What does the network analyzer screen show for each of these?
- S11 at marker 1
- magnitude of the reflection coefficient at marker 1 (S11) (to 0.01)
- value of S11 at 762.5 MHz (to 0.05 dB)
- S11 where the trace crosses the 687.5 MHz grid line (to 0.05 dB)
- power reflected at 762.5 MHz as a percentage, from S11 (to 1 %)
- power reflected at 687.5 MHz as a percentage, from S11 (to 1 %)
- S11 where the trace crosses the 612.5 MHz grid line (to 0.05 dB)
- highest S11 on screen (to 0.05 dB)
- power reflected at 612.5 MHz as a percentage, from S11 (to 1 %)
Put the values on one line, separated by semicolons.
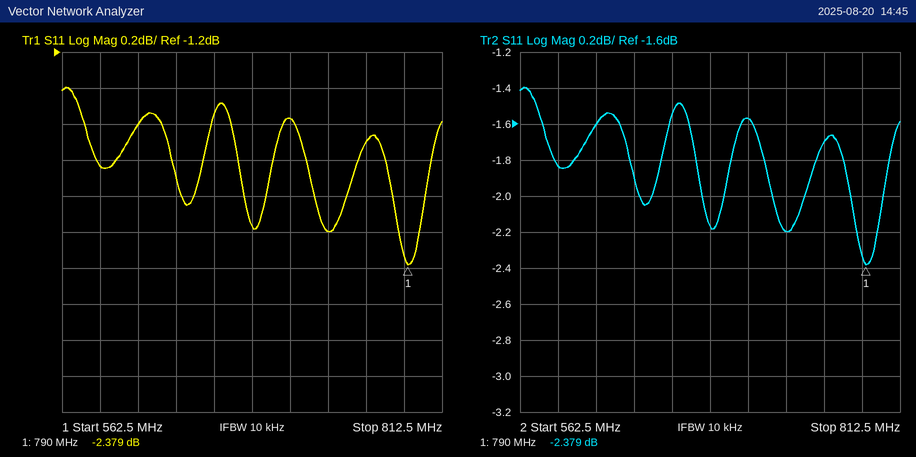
-2.379 dB; 0.76; -1.70 dB; -2.15 dB; 68 %; 61 %; -1.60 dB; -1.40 dB; 69 %
